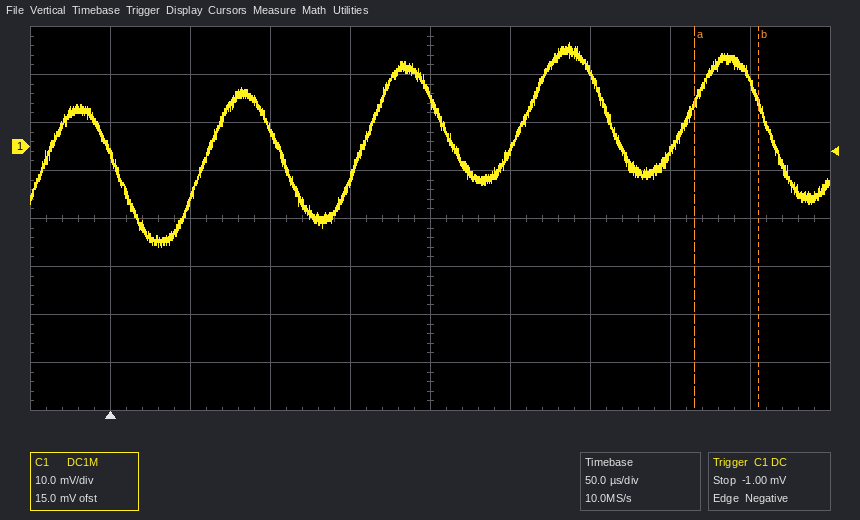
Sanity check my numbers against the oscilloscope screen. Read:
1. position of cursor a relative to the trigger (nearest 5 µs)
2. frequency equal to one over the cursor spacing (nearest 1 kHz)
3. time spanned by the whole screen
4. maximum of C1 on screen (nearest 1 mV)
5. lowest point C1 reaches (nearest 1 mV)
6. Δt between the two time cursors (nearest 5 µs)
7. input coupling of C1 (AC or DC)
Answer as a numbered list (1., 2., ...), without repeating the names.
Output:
1. +365 µs
2. 25 kHz
3. 500 µs
4. 22 mV
5. -21 mV
6. 40 µs
7. DC
